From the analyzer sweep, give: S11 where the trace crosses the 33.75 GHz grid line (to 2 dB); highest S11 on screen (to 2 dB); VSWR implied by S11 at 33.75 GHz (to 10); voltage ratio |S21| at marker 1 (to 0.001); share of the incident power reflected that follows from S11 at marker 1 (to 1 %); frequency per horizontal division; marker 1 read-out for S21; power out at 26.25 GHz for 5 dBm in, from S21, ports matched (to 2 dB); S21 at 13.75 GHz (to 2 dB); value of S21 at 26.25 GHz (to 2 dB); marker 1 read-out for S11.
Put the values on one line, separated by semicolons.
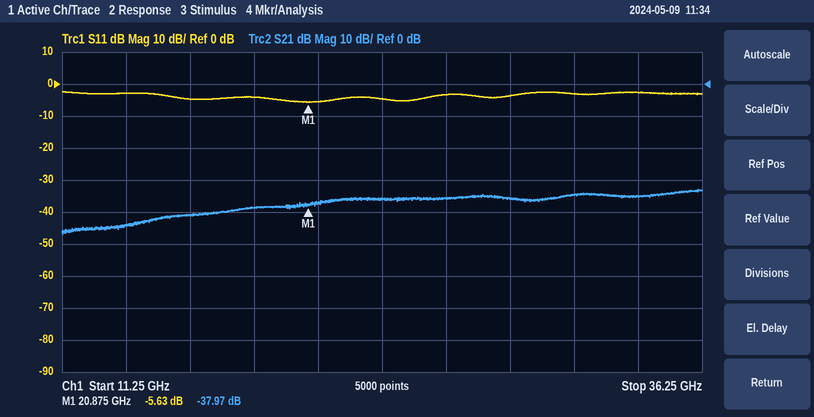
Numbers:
-2 dB; -2 dB; 10; 0.013; 27 %; 2.5 GHz; -37.97 dB; -30 dBm; -44 dB; -36 dB; -5.63 dB
